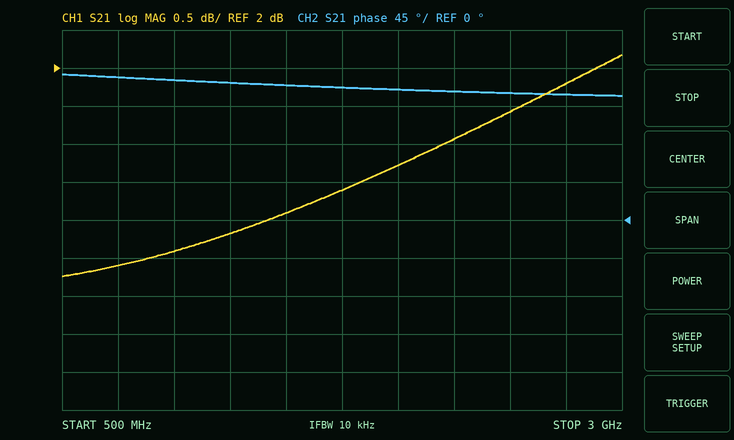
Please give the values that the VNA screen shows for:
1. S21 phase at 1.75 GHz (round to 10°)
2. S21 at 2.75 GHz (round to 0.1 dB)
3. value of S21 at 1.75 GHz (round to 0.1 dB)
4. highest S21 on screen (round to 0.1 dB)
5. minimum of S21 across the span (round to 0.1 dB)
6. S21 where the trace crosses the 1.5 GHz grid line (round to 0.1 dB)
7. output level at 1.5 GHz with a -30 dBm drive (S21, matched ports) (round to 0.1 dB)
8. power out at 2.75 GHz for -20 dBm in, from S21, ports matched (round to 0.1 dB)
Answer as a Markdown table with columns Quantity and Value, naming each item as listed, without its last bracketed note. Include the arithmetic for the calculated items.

| Quantity | Value |
|---|---|
| S21 phase at 1.75 GHz | 160° |
| S21 at 2.75 GHz | 1.8 dB |
| value of S21 at 1.75 GHz | 0.4 dB |
| highest S21 on screen | 2.2 dB |
| minimum of S21 across the span | -0.7 dB |
| S21 where the trace crosses the 1.5 GHz grid line | 0.1 dB |
| output level at 1.5 GHz with a -30 dBm drive (S21, matched ports) | -30 dBm + (0.1 dB) = -29.9 dBm |
| power out at 2.75 GHz for -20 dBm in, from S21, ports matched | -20 dBm + (1.8 dB) = -18.2 dBm |
